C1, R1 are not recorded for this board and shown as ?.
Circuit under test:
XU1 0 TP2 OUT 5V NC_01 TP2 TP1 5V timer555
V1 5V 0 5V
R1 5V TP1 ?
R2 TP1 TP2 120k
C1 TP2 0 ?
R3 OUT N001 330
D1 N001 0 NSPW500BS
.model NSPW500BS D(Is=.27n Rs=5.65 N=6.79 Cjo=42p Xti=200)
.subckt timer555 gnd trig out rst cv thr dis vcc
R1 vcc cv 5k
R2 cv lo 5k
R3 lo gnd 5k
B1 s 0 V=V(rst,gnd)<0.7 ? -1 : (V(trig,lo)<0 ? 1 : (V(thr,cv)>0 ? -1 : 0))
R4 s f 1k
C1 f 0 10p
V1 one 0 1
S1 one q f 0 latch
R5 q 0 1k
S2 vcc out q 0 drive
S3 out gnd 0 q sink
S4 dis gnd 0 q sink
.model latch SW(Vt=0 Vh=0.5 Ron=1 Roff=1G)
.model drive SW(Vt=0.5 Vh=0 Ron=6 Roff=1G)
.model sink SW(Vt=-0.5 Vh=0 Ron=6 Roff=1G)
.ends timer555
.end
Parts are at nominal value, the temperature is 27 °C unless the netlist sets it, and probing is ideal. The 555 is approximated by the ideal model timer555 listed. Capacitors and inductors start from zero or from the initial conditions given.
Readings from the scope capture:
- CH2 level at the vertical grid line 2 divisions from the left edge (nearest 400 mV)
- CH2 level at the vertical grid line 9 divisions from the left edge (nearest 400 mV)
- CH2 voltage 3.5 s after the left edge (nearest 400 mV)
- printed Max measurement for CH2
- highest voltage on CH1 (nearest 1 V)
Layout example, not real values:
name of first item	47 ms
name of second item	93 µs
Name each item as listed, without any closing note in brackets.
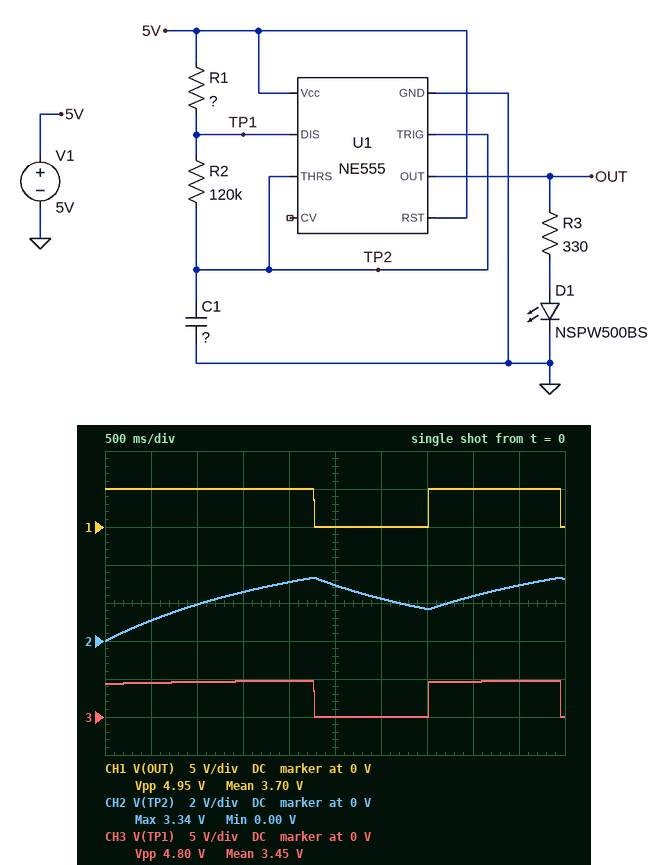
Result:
CH2 level at the vertical grid line 2 divisions from the left edge	2.0 V
CH2 level at the vertical grid line 9 divisions from the left edge	2.8 V
CH2 voltage 3.5 s after the left edge	1.6 V
printed Max measurement for CH2	3.34 V
highest voltage on CH1	5 V
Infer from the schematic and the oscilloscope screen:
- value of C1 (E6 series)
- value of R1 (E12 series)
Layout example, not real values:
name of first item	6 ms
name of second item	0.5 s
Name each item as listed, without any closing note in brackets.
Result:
value of C1	15 µF
value of R1	18 kΩ
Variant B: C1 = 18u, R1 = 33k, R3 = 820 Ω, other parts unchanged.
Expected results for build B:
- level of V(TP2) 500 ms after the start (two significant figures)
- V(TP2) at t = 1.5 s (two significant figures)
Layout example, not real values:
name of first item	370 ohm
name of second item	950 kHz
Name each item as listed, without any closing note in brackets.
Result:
level of V(TP2) 500 ms after the start	830 mV
V(TP2) at t = 1.5 s	2.1 V
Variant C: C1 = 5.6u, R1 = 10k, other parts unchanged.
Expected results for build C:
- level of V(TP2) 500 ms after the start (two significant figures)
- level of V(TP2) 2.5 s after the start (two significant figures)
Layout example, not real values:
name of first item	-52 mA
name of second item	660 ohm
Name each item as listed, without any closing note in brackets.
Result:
level of V(TP2) 500 ms after the start	2.5 V
level of V(TP2) 2.5 s after the start	2.7 V
